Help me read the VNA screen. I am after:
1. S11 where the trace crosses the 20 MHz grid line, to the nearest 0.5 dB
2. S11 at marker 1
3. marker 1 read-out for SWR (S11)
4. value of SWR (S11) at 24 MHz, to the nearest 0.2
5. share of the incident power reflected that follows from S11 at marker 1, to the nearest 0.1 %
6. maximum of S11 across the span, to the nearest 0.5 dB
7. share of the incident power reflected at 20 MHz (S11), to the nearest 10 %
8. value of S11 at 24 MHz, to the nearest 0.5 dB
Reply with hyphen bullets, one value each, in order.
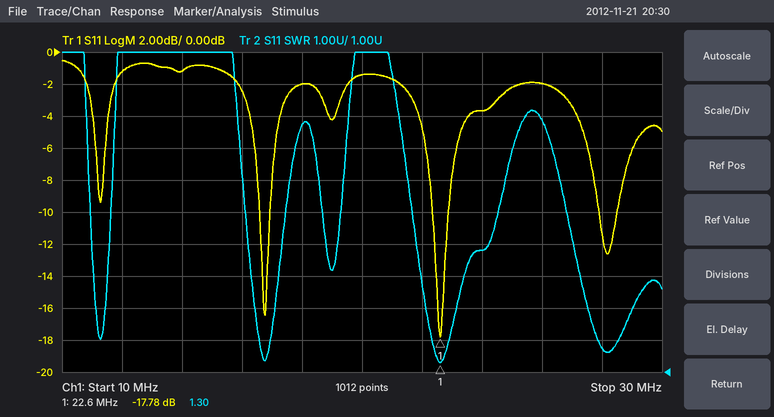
- -1.5 dB
- -17.78 dB
- 1.30
- 4.8
- 1.7 %
- -0.5 dB
- 70 %
- -3.5 dB
